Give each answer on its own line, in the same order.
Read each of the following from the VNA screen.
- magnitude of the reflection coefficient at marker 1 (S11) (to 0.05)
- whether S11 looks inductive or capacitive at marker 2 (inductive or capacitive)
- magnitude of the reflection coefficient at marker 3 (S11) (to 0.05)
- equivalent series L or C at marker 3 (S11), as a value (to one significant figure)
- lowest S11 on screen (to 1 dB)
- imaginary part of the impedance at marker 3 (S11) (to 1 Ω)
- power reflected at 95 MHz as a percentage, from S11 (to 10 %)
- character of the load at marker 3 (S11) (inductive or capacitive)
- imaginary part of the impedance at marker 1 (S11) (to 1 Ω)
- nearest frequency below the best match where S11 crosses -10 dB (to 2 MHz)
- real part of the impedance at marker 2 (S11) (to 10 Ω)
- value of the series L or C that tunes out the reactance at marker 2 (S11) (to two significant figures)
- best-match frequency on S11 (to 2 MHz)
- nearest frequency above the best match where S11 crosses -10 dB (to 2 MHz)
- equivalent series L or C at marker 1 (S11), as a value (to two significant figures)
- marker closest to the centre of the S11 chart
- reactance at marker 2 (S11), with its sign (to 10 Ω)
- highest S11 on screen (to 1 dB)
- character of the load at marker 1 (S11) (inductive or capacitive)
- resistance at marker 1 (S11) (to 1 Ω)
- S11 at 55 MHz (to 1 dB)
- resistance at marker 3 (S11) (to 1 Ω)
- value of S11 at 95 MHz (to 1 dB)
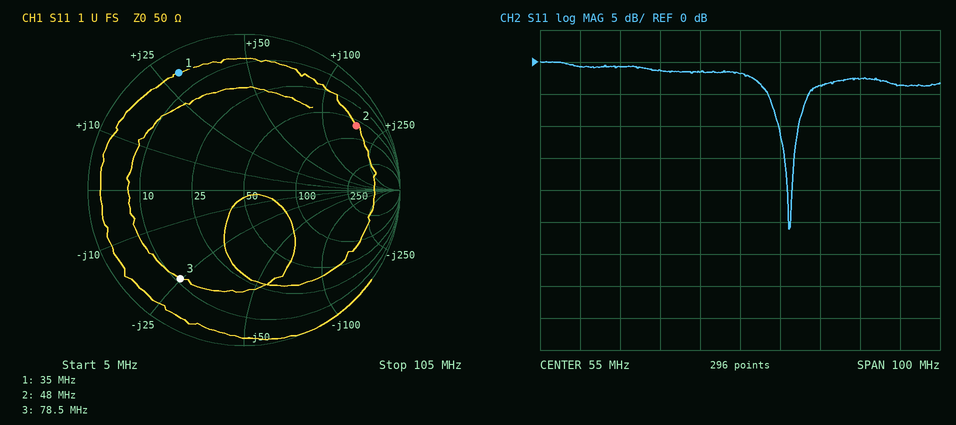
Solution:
0.85
inductive
0.70
80 pF
-26 dB
-25 Ω
40 %
capacitive
+29 Ω
64 MHz
60 Ω
20 pF
68 MHz
70 MHz
130 nH
marker 3
+170 Ω
0 dB
inductive
5 Ω
-2 dB
11 Ω
-4 dB
